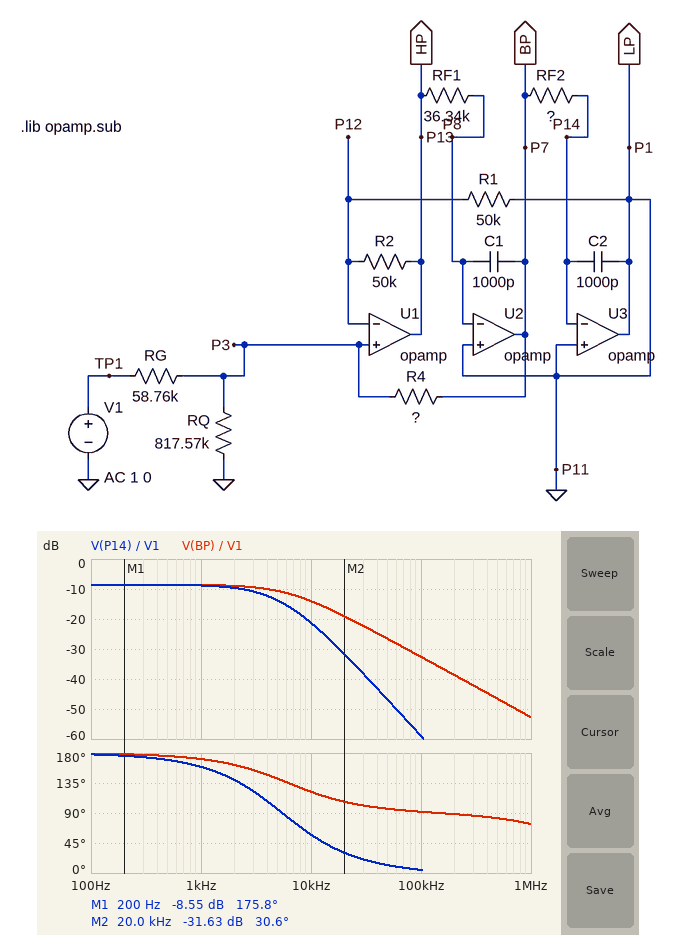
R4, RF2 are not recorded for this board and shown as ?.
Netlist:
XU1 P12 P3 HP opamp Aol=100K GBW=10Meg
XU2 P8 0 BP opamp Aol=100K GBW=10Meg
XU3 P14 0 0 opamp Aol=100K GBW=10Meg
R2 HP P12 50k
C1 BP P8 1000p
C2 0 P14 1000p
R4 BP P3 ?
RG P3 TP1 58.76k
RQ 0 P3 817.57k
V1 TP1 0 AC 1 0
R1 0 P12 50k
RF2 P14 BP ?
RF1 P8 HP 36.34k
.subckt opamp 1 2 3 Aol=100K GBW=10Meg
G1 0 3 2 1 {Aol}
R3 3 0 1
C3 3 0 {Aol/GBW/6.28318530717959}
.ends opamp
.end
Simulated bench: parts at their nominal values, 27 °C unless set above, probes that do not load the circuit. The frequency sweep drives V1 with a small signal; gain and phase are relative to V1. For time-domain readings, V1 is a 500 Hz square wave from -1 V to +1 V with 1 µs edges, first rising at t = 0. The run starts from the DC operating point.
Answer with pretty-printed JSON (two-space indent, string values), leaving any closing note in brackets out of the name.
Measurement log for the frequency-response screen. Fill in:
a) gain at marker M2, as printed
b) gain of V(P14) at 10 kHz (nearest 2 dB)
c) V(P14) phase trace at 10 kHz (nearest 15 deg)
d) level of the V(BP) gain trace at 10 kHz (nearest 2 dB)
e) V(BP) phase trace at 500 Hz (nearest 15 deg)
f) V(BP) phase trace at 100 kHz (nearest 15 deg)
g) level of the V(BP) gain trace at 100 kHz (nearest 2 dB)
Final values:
{
  "gain at marker M2, as printed": "-31.63 dB",
  "gain of V(P14) at 10 kHz": "-22 dB",
  "V(P14) phase trace at 10 kHz": "60 deg",
  "level of the V(BP) gain trace at 10 kHz": "-14 dB",
  "V(BP) phase trace at 500 Hz": "180 deg",
  "V(BP) phase trace at 100 kHz": "90 deg",
  "level of the V(BP) gain trace at 100 kHz": "-32 dB"
}
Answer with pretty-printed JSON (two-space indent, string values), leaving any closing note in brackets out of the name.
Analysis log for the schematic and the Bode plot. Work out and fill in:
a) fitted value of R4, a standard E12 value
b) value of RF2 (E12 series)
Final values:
{
  "fitted value of R4, a standard E12 value": "22 kΩ",
  "value of RF2": "33 kΩ"
}
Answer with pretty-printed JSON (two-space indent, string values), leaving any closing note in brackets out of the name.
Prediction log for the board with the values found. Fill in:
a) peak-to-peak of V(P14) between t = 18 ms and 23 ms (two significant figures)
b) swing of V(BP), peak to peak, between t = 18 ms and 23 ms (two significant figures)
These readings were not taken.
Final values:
{
  "peak-to-peak of V(P14) between t = 18 ms and 23 ms": "750 mV",
  "swing of V(BP), peak to peak, between t = 18 ms and 23 ms": "750 mV"
}
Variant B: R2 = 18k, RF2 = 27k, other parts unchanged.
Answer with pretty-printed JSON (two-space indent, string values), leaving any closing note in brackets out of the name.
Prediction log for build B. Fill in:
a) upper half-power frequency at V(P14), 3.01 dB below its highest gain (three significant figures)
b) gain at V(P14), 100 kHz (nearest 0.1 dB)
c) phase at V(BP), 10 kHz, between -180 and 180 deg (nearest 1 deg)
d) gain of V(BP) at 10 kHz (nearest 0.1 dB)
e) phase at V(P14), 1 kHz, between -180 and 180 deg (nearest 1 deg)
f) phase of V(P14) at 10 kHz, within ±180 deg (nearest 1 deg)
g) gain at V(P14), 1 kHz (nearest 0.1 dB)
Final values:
{
  "upper half-power frequency at V(P14), 3.01 dB below its highest gain": "3.16 kHz",
  "gain at V(P14), 100 kHz": "-60.6 dB",
  "phase at V(BP), 10 kHz, between -180 and 180 deg": "113 deg",
  "gain of V(BP) at 10 kHz": "-16.7 dB",
  "phase at V(P14), 1 kHz, between -180 and 180 deg": "157 deg",
  "phase of V(P14) at 10 kHz, within ±180 deg": "53 deg",
  "gain at V(P14), 1 kHz": "-8.9 dB"
}
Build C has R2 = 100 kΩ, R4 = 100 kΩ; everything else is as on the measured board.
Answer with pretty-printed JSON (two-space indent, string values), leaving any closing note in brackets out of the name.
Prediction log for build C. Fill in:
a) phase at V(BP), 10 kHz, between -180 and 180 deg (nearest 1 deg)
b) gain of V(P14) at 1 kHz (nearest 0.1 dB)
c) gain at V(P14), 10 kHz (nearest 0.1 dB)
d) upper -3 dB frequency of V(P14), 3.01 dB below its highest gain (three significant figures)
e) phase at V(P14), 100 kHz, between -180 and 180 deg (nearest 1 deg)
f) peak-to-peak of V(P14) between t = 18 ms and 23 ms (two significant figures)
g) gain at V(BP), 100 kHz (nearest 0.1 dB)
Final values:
{
  "phase at V(BP), 10 kHz, between -180 and 180 deg": "115 deg",
  "gain of V(P14) at 1 kHz": "4.2 dB",
  "gain at V(P14), 10 kHz": "-10.1 dB",
  "upper -3 dB frequency of V(P14), 3.01 dB below its highest gain": "3.05 kHz",
  "phase at V(P14), 100 kHz, between -180 and 180 deg": "3 deg",
  "peak-to-peak of V(P14) between t = 18 ms and 23 ms": "3.4 V",
  "gain at V(BP), 100 kHz": "-22.0 dB"
}
